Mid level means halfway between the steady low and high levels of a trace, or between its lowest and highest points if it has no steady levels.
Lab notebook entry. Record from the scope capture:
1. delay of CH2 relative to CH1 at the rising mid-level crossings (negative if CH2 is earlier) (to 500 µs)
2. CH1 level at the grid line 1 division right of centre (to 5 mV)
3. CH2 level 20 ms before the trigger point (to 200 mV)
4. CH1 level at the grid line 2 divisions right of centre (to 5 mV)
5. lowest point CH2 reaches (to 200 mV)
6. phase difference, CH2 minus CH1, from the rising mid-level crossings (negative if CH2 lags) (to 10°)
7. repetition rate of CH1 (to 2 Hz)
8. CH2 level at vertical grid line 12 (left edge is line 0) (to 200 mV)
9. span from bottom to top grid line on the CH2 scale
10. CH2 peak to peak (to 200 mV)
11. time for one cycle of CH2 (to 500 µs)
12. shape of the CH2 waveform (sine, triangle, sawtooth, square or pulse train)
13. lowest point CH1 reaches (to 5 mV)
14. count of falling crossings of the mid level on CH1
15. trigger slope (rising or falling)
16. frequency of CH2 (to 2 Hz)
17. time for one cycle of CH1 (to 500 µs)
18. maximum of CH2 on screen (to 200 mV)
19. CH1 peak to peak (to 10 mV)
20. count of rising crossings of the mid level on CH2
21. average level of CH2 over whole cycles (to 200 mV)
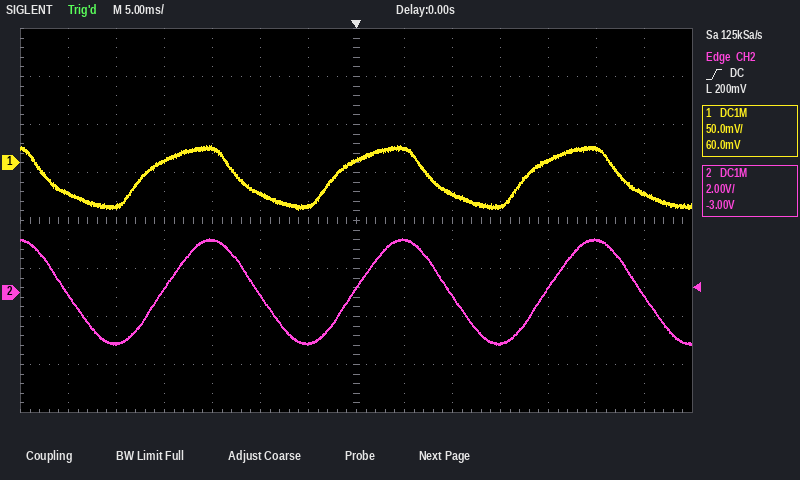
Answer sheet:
+2.0 ms
15 mV
200 mV
-30 mV
-2.2 V
-40°
50 Hz
2.2 V
16 V
4.4 V
20.0 ms
sine
-50 mV
4
rising
50 Hz
20.0 ms
2.2 V
70 mV
3
0.0 V
